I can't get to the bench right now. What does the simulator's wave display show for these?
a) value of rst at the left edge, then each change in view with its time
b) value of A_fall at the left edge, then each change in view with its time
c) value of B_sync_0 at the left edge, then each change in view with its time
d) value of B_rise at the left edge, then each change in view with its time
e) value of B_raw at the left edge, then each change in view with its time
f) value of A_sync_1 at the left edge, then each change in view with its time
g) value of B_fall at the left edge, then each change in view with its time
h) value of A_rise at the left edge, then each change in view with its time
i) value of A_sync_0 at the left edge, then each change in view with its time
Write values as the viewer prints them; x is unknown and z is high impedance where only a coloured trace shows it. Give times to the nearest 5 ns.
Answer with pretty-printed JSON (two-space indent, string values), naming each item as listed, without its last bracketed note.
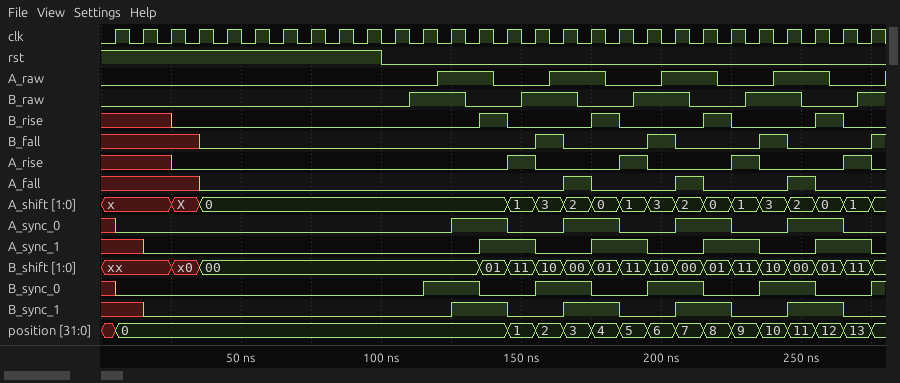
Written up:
{
  "value of rst at the left edge, then each change in view with its time": "1, 0 at 100 ns",
  "value of A_fall at the left edge, then each change in view with its time": "x, 0 at 35 ns, 1 at 165 ns, 0 at 175 ns, 1 at 205 ns, 0 at 215 ns, 1 at 245 ns, 0 at 255 ns",
  "value of B_sync_0 at the left edge, then each change in view with its time": "x, 0 at 5 ns, 1 at 115 ns, 0 at 135 ns, 1 at 155 ns, 0 at 175 ns, 1 at 195 ns, 0 at 215 ns, 1 at 235 ns, 0 at 255 ns, 1 at 275 ns",
  "value of B_rise at the left edge, then each change in view with its time": "x, 0 at 25 ns, 1 at 135 ns, 0 at 145 ns, 1 at 175 ns, 0 at 185 ns, 1 at 215 ns, 0 at 225 ns, 1 at 255 ns, 0 at 265 ns",
  "value of B_raw at the left edge, then each change in view with its time": "0, 1 at 110 ns, 0 at 130 ns, 1 at 150 ns, 0 at 170 ns, 1 at 190 ns, 0 at 210 ns, 1 at 230 ns, 0 at 250 ns, 1 at 270 ns",
  "value of A_sync_1 at the left edge, then each change in view with its time": "x, 0 at 15 ns, 1 at 135 ns, 0 at 155 ns, 1 at 175 ns, 0 at 195 ns, 1 at 215 ns, 0 at 235 ns, 1 at 255 ns, 0 at 275 ns",
  "value of B_fall at the left edge, then each change in view with its time": "x, 0 at 35 ns, 1 at 155 ns, 0 at 165 ns, 1 at 195 ns, 0 at 205 ns, 1 at 235 ns, 0 at 245 ns, 1 at 275 ns",
  "value of A_rise at the left edge, then each change in view with its time": "x, 0 at 25 ns, 1 at 145 ns, 0 at 155 ns, 1 at 185 ns, 0 at 195 ns, 1 at 225 ns, 0 at 235 ns, 1 at 265 ns, 0 at 275 ns",
  "value of A_sync_0 at the left edge, then each change in view with its time": "x, 0 at 5 ns, 1 at 125 ns, 0 at 145 ns, 1 at 165 ns, 0 at 185 ns, 1 at 205 ns, 0 at 225 ns, 1 at 245 ns, 0 at 265 ns"
}
